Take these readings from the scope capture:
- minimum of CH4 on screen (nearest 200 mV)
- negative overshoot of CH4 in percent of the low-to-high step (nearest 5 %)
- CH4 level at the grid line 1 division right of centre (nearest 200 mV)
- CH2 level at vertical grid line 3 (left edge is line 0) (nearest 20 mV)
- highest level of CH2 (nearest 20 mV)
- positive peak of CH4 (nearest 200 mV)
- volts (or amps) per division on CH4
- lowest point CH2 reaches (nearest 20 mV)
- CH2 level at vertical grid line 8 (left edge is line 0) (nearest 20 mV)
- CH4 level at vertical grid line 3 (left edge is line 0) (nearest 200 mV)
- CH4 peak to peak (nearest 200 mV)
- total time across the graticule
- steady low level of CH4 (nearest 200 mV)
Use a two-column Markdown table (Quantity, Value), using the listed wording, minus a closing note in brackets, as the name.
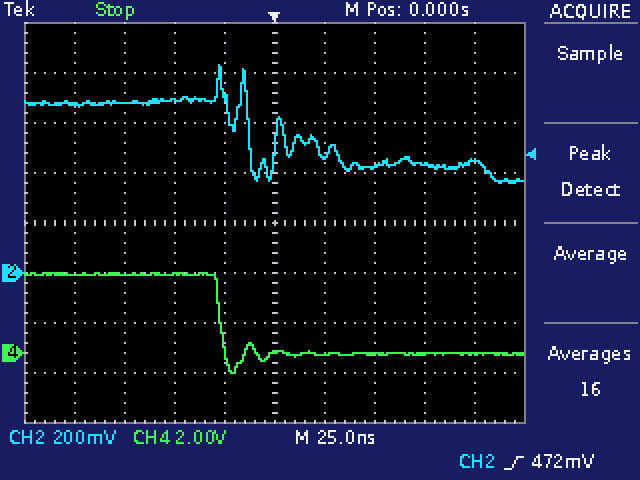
| Quantity | Value |
|---|---|
| minimum of CH4 on screen | -800 mV |
| negative overshoot of CH4 in percent of the low-to-high step | 25 % |
| CH4 level at the grid line 1 division right of centre | 0.0 V |
| CH2 level at vertical grid line 3 (left edge is line 0) | 700 mV |
| highest level of CH2 | 840 mV |
| positive peak of CH4 | 3.2 V |
| volts (or amps) per division on CH4 | 2 V |
| lowest point CH2 reaches | 360 mV |
| CH2 level at vertical grid line 8 (left edge is line 0) | 440 mV |
| CH4 level at vertical grid line 3 (left edge is line 0) | 3.2 V |
| CH4 peak to peak | 4.0 V |
| total time across the graticule | 250 ns |
| steady low level of CH4 | 0.0 V |
